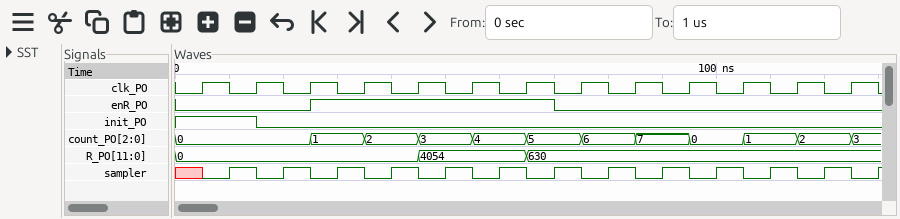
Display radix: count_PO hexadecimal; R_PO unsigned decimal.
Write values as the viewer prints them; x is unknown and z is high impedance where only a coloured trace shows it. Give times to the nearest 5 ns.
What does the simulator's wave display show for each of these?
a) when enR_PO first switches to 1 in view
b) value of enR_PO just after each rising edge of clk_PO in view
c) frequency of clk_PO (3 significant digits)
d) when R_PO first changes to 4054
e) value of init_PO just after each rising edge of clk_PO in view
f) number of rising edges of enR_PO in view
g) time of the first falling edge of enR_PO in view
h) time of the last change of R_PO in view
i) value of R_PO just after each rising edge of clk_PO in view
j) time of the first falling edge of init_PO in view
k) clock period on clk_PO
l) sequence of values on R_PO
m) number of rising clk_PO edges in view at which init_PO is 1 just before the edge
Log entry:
25 ns
0 0 1 1 1 1 1 0 0 0 0 0 0
100 MHz
45 ns
1 0 0 0 0 0 0 0 0 0 0 0 0
1
70 ns
65 ns
0, 0, 0, 0, 4054, 4054, 630, 630, 630, 630, 630, 630, 630
15 ns
10 ns
0, 4054, 630
2
